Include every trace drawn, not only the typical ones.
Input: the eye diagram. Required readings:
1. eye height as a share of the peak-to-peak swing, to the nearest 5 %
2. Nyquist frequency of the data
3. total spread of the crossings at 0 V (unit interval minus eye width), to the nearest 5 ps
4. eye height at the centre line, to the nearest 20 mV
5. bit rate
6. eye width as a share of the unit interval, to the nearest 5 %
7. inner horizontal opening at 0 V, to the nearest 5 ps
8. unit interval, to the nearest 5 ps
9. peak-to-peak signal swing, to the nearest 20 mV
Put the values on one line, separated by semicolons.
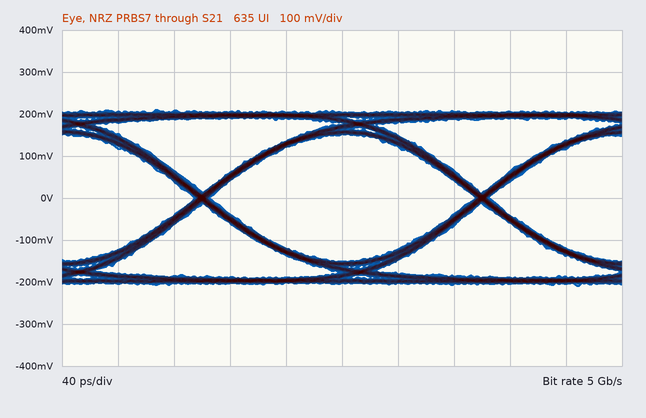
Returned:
70 %; 2.5 GHz; 10 ps; 300 mV; 5 Gb/s; 95 %; 190 ps; 200 ps; 420 mV
